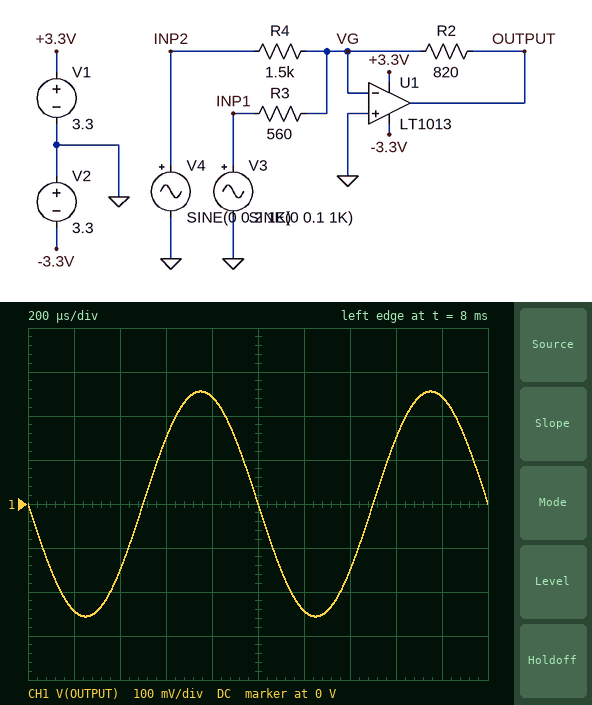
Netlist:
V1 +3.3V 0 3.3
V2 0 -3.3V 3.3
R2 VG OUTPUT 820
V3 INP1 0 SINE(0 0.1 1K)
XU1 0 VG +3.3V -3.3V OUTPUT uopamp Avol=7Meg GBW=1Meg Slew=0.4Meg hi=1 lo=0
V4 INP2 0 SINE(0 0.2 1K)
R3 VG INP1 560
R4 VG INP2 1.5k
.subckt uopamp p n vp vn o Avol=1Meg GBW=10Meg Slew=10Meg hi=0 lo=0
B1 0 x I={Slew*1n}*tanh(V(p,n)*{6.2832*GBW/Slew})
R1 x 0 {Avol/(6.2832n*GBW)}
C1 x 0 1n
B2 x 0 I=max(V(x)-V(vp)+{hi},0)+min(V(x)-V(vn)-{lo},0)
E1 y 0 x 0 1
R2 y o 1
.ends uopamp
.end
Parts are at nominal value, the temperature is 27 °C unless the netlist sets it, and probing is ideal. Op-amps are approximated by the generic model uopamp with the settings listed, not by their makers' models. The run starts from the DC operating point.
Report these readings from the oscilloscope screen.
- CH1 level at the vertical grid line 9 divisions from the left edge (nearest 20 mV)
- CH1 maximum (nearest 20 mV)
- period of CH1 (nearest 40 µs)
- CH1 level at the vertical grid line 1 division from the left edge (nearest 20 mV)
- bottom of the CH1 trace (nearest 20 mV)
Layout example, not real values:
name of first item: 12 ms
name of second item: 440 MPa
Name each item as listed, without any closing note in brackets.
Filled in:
CH1 level at the vertical grid line 9 divisions from the left edge: 240 mV
CH1 maximum: 260 mV
period of CH1: 1.00 ms
CH1 level at the vertical grid line 1 division from the left edge: -240 mV
bottom of the CH1 trace: -260 mV
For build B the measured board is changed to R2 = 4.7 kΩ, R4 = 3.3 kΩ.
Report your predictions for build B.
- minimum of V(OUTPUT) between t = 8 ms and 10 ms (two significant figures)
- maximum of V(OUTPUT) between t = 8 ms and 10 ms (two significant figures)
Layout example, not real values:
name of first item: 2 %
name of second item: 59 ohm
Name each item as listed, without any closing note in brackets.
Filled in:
minimum of V(OUTPUT) between t = 8 ms and 10 ms: -1.1 V
maximum of V(OUTPUT) between t = 8 ms and 10 ms: 1.1 V
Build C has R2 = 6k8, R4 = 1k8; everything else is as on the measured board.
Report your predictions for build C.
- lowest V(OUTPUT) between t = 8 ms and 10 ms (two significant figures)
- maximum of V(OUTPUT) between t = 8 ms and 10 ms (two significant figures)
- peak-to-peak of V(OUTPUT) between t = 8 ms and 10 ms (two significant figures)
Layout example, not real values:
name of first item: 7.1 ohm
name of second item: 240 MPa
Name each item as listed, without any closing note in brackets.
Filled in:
lowest V(OUTPUT) between t = 8 ms and 10 ms: -2.0 V
maximum of V(OUTPUT) between t = 8 ms and 10 ms: 2.0 V
peak-to-peak of V(OUTPUT) between t = 8 ms and 10 ms: 3.9 V
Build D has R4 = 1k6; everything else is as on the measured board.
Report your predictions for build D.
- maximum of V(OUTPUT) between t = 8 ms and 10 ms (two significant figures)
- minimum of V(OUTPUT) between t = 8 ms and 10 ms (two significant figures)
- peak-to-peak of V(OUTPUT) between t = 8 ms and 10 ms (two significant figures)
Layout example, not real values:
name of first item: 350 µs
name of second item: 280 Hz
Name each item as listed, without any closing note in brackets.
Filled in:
maximum of V(OUTPUT) between t = 8 ms and 10 ms: 250 mV
minimum of V(OUTPUT) between t = 8 ms and 10 ms: -250 mV
peak-to-peak of V(OUTPUT) between t = 8 ms and 10 ms: 500 mV
